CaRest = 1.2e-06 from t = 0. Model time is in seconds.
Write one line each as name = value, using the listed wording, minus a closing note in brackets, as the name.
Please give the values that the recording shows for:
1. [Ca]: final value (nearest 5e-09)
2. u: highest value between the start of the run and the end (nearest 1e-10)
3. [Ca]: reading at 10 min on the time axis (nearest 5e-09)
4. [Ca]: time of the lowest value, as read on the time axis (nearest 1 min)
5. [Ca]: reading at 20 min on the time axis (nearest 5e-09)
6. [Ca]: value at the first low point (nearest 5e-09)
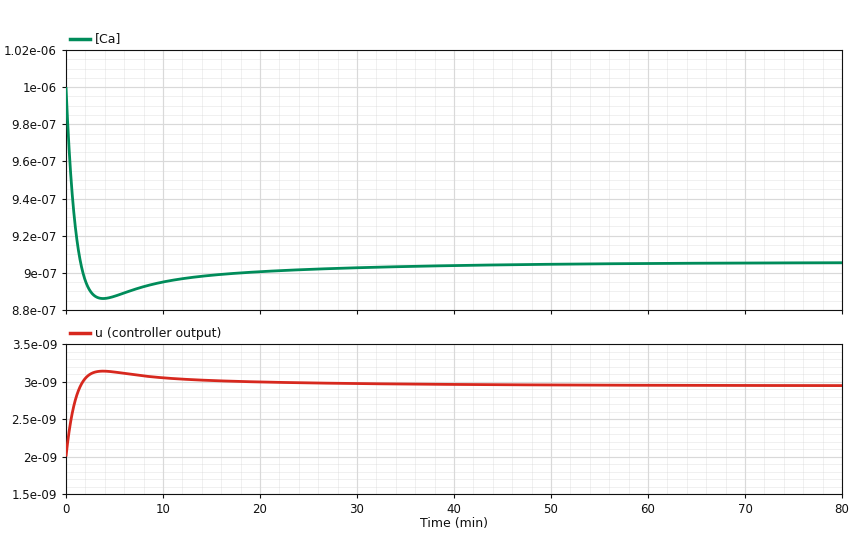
[Ca]: final value = 0.000000905
u: highest value between the start of the run and the end = 0.0000000031
[Ca]: reading at 10 min on the time axis = 0.000000895
[Ca]: time of the lowest value, as read on the time axis = 4 min
[Ca]: reading at 20 min on the time axis = 0.000000900
[Ca]: value at the first low point = 0.000000885
